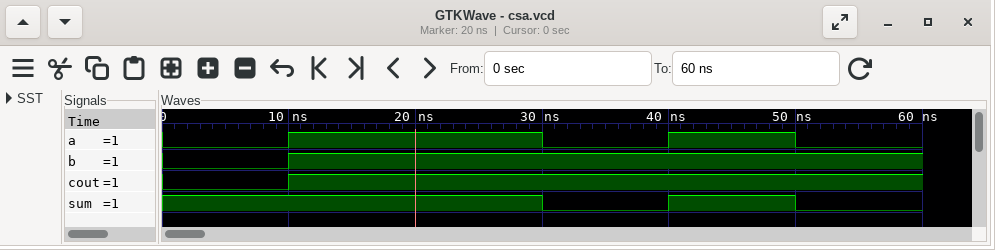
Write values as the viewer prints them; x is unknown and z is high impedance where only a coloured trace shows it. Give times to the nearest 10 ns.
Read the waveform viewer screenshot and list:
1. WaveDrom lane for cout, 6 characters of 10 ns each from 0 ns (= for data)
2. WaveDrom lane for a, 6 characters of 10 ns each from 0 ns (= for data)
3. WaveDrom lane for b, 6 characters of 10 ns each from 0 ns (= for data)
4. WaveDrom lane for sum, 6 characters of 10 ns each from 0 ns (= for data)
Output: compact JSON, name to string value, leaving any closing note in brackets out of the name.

{"WaveDrom lane for cout, 6 characters of 10 ns each from 0 ns": "{name: 'cout', wave: '01....'}", "WaveDrom lane for a, 6 characters of 10 ns each from 0 ns": "{name: 'a', wave: '01.010'}", "WaveDrom lane for b, 6 characters of 10 ns each from 0 ns": "{name: 'b', wave: '01....'}", "WaveDrom lane for sum, 6 characters of 10 ns each from 0 ns": "{name: 'sum', wave: '1..010'}"}
